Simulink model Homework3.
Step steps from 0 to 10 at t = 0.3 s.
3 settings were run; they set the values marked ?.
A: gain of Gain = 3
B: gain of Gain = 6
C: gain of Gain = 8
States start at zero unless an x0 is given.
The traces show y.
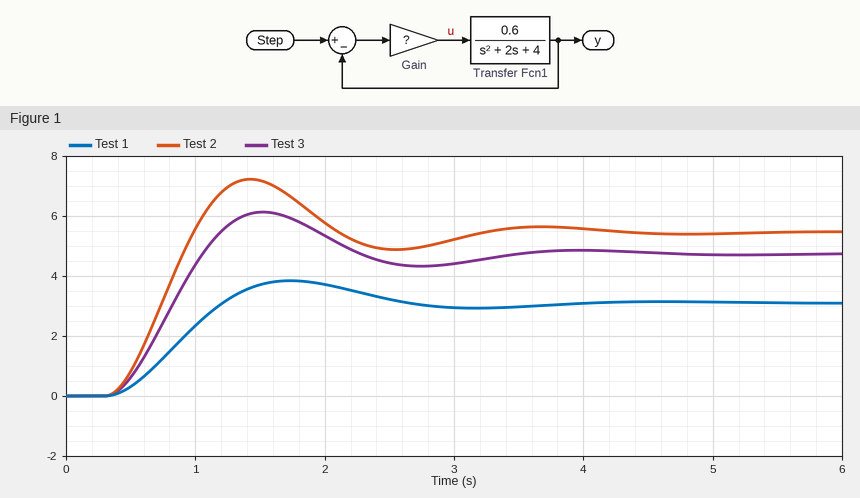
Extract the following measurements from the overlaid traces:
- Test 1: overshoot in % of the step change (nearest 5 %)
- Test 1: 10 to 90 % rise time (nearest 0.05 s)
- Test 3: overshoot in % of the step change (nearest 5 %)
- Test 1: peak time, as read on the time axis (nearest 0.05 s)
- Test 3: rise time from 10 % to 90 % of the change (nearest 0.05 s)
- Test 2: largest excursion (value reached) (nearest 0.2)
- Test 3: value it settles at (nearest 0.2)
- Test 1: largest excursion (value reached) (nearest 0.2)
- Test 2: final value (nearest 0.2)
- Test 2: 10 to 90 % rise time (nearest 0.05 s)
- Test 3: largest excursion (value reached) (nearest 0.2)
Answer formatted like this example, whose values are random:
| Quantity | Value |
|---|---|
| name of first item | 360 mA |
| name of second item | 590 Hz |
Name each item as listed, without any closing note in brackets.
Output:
| Quantity | Value |
|---|---|
| Test 1: overshoot in % of the step change | 25 % |
| Test 1: 10 to 90 % rise time | 0.60 s |
| Test 3: overshoot in % of the step change | 30 % |
| Test 1: peak time, as read on the time axis | 1.75 s |
| Test 3: rise time from 10 % to 90 % of the change | 0.50 s |
| Test 2: largest excursion (value reached) | 7.2 |
| Test 3: value it settles at | 4.8 |
| Test 1: largest excursion (value reached) | 3.8 |
| Test 2: final value | 5.4 |
| Test 2: 10 to 90 % rise time | 0.45 s |
| Test 3: largest excursion (value reached) | 6.2 |
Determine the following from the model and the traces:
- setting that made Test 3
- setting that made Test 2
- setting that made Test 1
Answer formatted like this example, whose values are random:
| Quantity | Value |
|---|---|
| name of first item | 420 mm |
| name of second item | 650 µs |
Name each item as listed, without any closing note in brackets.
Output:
| Quantity | Value |
|---|---|
| setting that made Test 3 | B |
| setting that made Test 2 | C |
| setting that made Test 1 | A |
